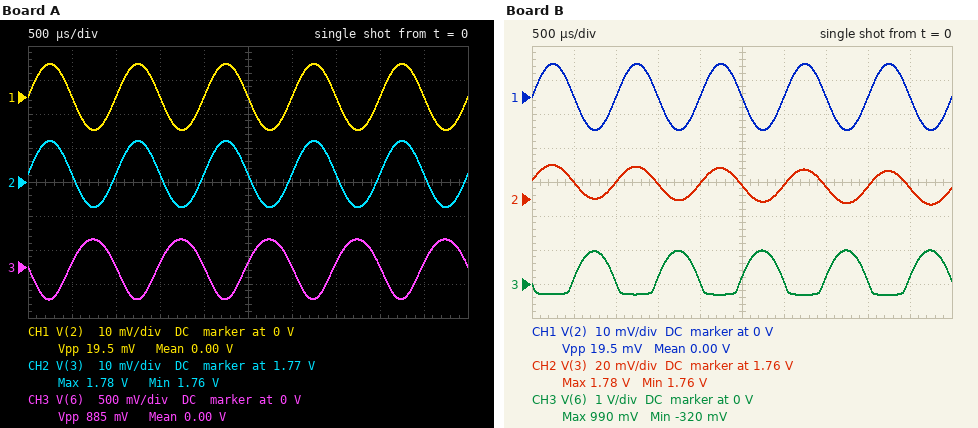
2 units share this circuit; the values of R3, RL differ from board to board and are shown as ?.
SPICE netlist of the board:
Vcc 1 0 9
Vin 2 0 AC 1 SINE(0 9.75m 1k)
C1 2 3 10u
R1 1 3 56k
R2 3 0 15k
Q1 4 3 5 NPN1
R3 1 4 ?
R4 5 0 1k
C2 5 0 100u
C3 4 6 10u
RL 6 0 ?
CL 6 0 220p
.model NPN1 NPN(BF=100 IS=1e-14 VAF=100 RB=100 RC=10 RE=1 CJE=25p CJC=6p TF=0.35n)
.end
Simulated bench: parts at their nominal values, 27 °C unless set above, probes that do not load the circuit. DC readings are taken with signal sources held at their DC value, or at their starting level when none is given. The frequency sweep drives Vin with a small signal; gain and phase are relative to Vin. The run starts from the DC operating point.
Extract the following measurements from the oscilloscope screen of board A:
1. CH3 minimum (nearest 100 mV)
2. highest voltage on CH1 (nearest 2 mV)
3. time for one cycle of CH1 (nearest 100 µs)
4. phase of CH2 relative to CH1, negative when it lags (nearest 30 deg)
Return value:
-500 mV
10 mV
1.0 ms
0 deg
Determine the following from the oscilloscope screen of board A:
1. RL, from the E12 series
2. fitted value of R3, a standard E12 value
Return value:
1.5 kΩ
5.6 kΩ
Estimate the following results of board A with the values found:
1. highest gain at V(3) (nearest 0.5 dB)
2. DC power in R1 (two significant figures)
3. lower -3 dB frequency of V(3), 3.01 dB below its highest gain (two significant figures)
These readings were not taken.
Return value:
0 dB
930 µW
1.7 Hz
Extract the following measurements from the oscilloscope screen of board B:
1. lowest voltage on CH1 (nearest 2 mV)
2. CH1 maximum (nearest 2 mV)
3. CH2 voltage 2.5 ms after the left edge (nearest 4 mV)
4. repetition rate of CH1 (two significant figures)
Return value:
-10 mV
10 mV
1.768 V
1.0 kHz
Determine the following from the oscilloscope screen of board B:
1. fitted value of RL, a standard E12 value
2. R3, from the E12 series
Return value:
4.7 kΩ
6.8 kΩ
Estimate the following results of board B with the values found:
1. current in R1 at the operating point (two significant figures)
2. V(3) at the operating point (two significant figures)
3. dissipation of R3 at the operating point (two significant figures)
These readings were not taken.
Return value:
130 µA
1.8 V
8.2 mW
